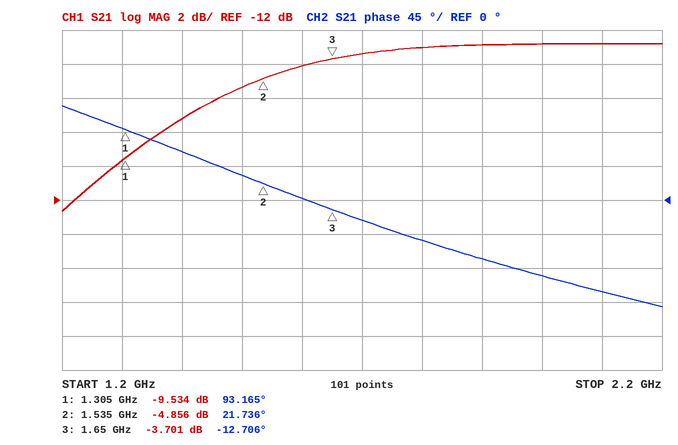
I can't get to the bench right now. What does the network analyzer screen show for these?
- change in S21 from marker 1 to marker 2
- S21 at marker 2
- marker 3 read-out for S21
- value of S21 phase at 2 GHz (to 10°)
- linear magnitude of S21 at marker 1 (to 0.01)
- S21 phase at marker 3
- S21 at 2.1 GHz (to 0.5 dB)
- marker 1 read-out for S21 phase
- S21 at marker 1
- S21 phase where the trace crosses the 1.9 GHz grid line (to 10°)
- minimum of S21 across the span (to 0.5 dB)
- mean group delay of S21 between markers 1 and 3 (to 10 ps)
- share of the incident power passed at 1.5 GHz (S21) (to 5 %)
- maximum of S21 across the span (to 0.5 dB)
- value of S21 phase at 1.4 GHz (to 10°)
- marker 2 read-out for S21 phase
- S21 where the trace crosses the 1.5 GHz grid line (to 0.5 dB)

4.678 dB
-4.856 dB
-3.701 dB
-100°
0.33
-12.706°
-3.0 dB
93.165°
-9.534 dB
-80°
-12.5 dB
850 ps
30 %
-3.0 dB
60°
21.736°
-5.5 dB
